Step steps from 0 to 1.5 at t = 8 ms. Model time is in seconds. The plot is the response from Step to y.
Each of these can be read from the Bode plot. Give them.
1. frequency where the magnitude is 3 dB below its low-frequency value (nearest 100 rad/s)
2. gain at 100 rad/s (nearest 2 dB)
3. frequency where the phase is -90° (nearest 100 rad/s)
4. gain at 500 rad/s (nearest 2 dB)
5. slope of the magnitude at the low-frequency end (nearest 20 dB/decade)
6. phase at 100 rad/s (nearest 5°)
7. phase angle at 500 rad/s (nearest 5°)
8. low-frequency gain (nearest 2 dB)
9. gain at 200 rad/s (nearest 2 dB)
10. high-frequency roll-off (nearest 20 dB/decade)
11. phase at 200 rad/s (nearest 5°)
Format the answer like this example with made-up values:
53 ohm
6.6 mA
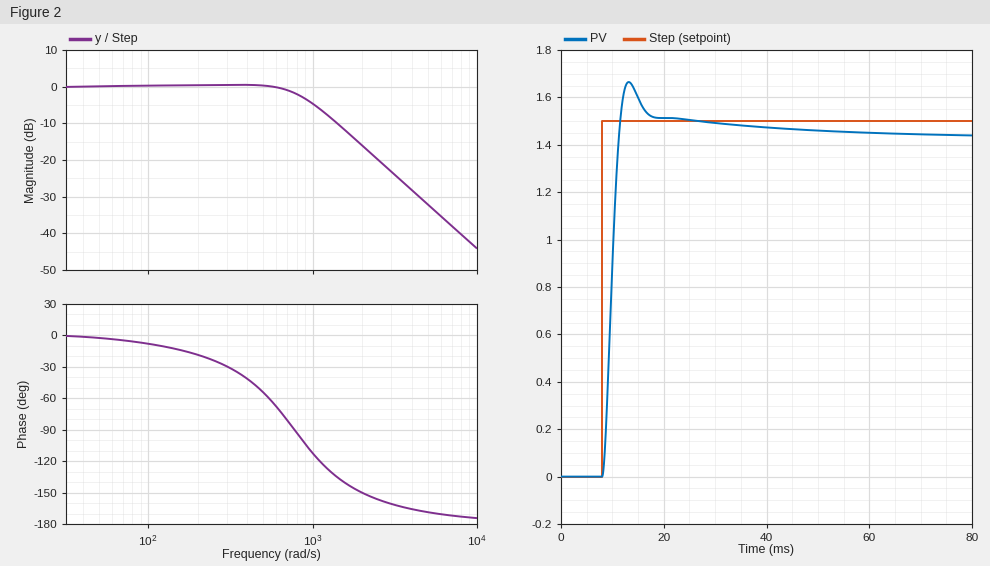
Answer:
900 rad/s
0 dB
800 rad/s
0 dB
0 dB/decade
-10°
-55°
0 dB
0 dB
-40 dB/decade
-20°
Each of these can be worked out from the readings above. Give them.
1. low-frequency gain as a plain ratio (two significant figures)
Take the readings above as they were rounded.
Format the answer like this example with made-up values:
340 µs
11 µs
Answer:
1.0
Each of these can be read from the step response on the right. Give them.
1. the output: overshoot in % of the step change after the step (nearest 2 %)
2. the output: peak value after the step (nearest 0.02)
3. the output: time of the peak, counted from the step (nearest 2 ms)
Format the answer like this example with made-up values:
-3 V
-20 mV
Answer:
16 %
1.66
6 ms
